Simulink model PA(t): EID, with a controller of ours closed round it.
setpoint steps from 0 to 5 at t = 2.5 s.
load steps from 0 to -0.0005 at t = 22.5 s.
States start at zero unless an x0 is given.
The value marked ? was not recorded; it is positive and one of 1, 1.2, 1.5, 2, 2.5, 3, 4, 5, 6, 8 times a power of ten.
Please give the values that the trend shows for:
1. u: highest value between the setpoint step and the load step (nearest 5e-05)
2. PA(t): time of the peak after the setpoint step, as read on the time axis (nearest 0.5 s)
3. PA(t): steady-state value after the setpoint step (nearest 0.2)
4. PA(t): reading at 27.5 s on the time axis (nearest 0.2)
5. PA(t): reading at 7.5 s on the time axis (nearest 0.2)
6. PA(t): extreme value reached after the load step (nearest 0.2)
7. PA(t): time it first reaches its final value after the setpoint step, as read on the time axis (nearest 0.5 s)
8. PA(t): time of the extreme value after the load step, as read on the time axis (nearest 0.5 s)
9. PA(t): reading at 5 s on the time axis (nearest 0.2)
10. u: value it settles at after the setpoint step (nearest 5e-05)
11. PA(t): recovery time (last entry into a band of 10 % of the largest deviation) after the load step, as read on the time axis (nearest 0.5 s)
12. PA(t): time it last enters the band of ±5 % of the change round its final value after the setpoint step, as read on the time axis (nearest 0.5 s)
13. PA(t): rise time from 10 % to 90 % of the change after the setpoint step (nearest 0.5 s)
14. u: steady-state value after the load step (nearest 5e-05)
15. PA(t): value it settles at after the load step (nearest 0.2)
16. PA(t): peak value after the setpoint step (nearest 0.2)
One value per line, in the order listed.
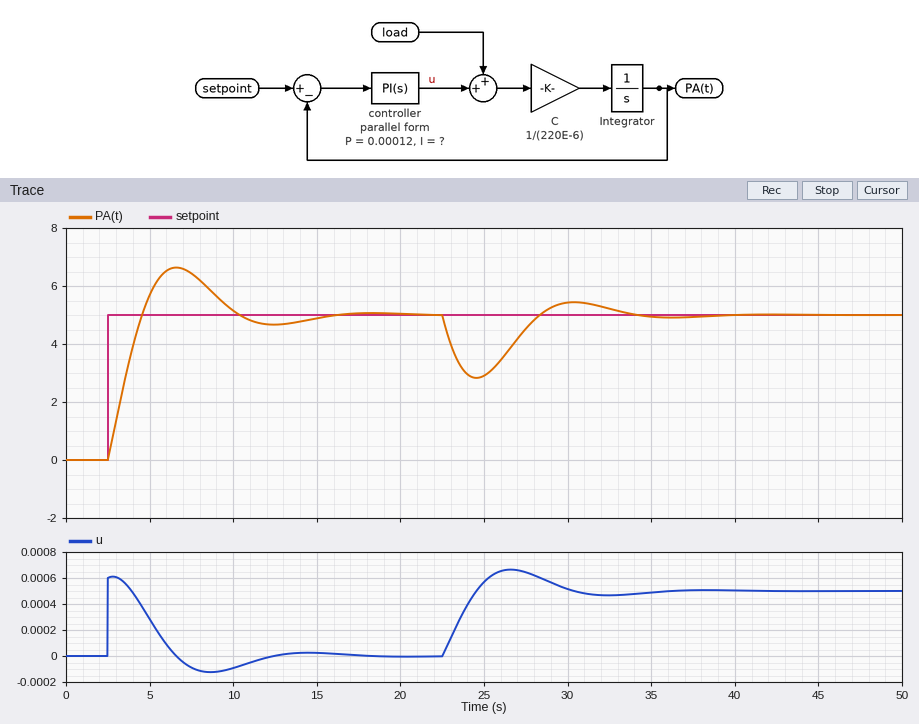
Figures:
0.00060
6.5 s
5.0
4.6
6.4
2.8
4.5 s
24.5 s
5.6
0.00000
32.5 s
14.0 s
1.5 s
0.00050
5.0
6.6
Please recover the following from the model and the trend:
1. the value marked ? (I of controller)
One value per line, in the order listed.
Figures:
8e-05
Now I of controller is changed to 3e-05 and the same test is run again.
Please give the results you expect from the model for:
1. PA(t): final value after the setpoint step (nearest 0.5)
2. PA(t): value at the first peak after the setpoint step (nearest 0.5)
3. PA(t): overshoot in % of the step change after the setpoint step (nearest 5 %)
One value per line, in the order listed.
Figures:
5.0
6.0
20 %
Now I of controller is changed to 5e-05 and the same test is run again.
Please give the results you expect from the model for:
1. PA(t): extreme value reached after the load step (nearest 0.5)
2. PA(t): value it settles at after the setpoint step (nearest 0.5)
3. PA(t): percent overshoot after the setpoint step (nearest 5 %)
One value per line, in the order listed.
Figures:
2.5
5.0
25 %
